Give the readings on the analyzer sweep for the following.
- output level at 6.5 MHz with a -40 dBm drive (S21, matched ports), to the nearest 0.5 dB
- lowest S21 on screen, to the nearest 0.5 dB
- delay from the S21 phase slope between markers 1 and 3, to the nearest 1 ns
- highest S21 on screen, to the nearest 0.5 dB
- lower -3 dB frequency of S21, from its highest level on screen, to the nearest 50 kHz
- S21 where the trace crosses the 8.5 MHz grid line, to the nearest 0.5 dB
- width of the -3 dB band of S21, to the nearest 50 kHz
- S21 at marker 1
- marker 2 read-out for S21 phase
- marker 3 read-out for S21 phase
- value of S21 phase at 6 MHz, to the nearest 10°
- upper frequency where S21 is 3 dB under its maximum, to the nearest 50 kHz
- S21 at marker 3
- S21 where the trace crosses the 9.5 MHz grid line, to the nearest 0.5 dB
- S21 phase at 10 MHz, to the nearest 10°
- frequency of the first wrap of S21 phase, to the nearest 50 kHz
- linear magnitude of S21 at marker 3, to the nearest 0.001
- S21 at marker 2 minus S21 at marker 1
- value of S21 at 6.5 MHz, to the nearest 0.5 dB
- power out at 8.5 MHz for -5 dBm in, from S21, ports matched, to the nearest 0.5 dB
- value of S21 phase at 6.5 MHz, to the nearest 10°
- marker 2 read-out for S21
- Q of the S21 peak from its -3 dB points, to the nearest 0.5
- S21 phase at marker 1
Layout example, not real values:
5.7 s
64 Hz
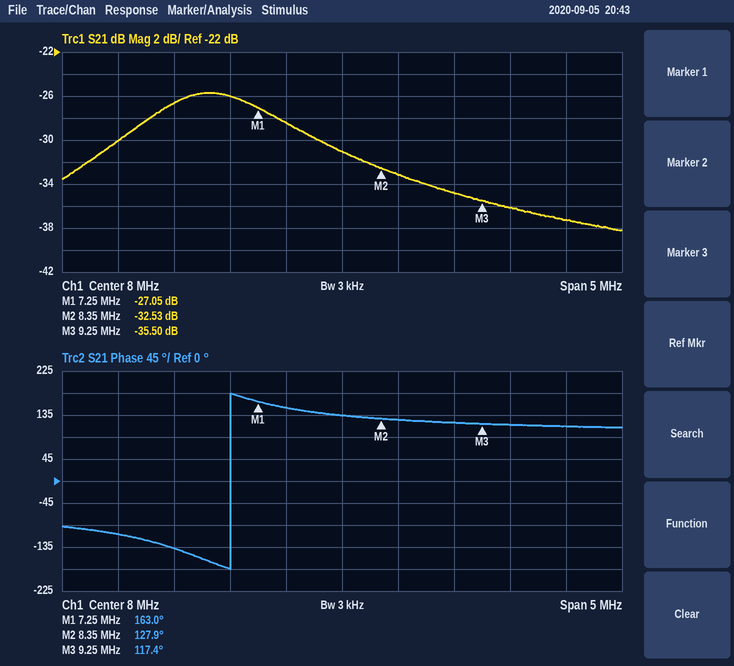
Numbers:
-66.5 dBm
-38.0 dB
63 ns
-25.5 dB
6.20 MHz
-33.0 dB
1.35 MHz
-27.05 dB
127.9°
117.4°
-110°
7.55 MHz
-35.50 dB
-36.0 dB
110°
7.00 MHz
0.017
-5.48 dB
-26.5 dB
-38.0 dBm
-140°
-32.53 dB
5.0
163.0°
